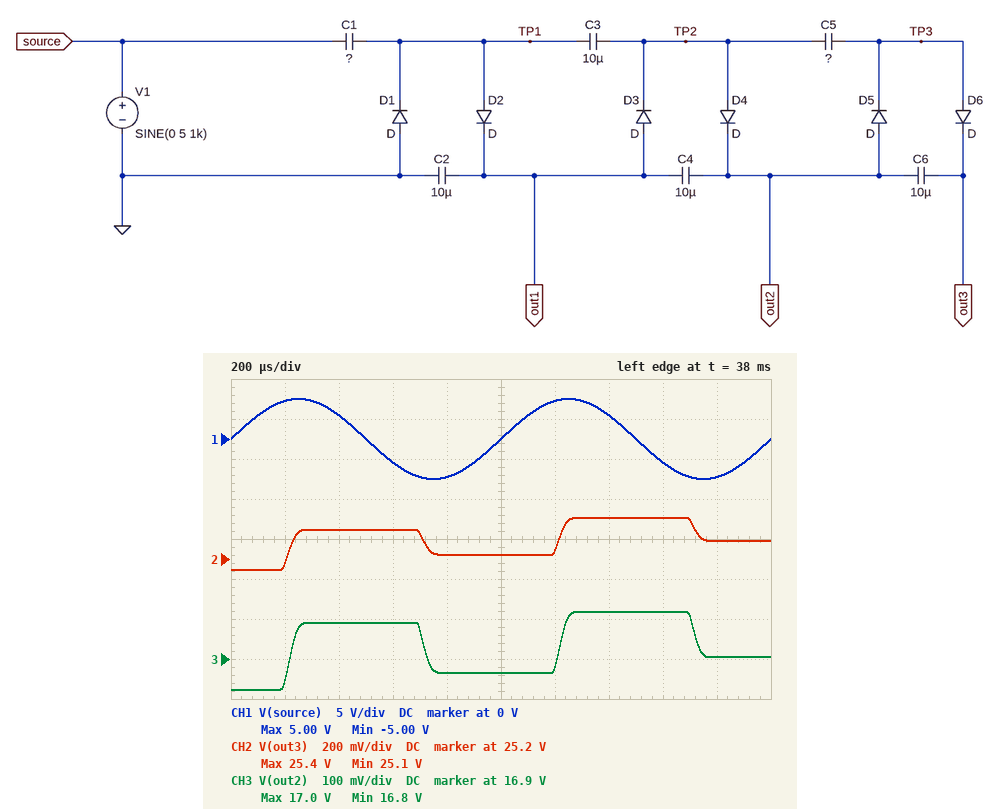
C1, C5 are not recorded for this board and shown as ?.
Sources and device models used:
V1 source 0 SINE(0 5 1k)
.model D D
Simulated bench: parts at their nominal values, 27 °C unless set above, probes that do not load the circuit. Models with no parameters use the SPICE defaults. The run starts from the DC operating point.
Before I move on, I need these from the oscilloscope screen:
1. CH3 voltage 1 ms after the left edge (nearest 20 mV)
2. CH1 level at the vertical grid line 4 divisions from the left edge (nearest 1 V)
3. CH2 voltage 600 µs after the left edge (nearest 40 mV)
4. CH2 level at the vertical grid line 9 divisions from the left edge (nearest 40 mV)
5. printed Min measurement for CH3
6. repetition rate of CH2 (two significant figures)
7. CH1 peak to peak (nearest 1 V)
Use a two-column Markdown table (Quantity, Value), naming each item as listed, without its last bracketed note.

| Quantity | Value |
|---|---|
| CH3 voltage 1 ms after the left edge | 16.86 V |
| CH1 level at the vertical grid line 4 divisions from the left edge | -5 V |
| CH2 voltage 600 µs after the left edge | 25.36 V |
| CH2 level at the vertical grid line 9 divisions from the left edge | 25.28 V |
| printed Min measurement for CH3 | 16.8 V |
| repetition rate of CH2 | 1.0 kHz |
| CH1 peak to peak | 10 V |
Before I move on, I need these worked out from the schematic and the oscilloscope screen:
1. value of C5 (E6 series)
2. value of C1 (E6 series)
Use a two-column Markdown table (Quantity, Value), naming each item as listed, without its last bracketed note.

| Quantity | Value |
|---|---|
| value of C5 | 3.3 µF |
| value of C1 | 15 µF |
